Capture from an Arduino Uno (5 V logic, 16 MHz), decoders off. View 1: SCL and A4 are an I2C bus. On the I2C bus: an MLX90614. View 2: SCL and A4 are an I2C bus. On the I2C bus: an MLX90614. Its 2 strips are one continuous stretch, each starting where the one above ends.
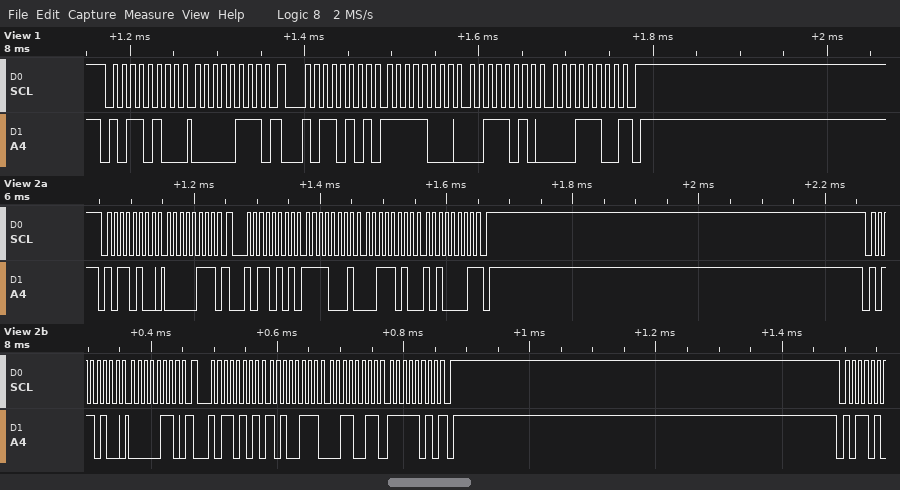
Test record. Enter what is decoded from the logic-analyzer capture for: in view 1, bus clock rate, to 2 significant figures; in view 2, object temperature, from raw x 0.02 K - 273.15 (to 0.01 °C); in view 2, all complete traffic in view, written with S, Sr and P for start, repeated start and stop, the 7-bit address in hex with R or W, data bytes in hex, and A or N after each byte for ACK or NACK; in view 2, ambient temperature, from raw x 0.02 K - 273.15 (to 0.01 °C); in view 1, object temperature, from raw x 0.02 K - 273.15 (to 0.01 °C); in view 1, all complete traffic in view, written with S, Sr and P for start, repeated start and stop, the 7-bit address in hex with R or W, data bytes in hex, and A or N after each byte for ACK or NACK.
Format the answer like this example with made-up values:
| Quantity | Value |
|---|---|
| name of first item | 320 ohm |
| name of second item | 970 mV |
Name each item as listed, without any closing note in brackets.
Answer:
| Quantity | Value |
|---|---|
| in view 1, bus clock rate, to 2 significant figures | 100 kHz |
| in view 2, object temperature, from raw x 0.02 K - 273.15 | 28.63 °C |
| in view 2, all complete traffic in view, written with S, Sr and P for start, repeated start and stop, the 7-bit address in hex with R or W, data bytes in hex, and A or N after each byte for ACK or NACK | S 5AW A 07 A Sr 5AR A F1 A 3A A A1 N P S 5AW A 06 A Sr 5AR A A7 A 33 A FA N P |
| in view 2, ambient temperature, from raw x 0.02 K - 273.15 | -8.69 °C |
| in view 1, object temperature, from raw x 0.02 K - 273.15 | 28.77 °C |
| in view 1, all complete traffic in view, written with S, Sr and P for start, repeated start and stop, the 7-bit address in hex with R or W, data bytes in hex, and A or N after each byte for ACK or NACK | S 5AW A 07 A Sr 5AR A F8 A 3A A 1C N P |
